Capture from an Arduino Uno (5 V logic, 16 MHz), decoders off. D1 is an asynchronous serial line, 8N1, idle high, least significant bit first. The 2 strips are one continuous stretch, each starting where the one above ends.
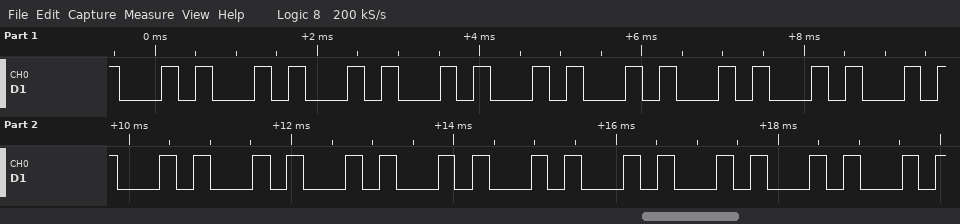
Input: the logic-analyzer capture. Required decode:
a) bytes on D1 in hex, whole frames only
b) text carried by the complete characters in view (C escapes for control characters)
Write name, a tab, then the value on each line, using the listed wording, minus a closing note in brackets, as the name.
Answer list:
bytes on D1 in hex, whole frames only	0x30 0x30 0x30 0x30 0x30 0x30 0x30 0x30 0x30 0x30 0x30 0x30 0x30 0x30 0x30 0x30 0x30 0x30
text carried by the complete characters in view	"000000000000000000"
